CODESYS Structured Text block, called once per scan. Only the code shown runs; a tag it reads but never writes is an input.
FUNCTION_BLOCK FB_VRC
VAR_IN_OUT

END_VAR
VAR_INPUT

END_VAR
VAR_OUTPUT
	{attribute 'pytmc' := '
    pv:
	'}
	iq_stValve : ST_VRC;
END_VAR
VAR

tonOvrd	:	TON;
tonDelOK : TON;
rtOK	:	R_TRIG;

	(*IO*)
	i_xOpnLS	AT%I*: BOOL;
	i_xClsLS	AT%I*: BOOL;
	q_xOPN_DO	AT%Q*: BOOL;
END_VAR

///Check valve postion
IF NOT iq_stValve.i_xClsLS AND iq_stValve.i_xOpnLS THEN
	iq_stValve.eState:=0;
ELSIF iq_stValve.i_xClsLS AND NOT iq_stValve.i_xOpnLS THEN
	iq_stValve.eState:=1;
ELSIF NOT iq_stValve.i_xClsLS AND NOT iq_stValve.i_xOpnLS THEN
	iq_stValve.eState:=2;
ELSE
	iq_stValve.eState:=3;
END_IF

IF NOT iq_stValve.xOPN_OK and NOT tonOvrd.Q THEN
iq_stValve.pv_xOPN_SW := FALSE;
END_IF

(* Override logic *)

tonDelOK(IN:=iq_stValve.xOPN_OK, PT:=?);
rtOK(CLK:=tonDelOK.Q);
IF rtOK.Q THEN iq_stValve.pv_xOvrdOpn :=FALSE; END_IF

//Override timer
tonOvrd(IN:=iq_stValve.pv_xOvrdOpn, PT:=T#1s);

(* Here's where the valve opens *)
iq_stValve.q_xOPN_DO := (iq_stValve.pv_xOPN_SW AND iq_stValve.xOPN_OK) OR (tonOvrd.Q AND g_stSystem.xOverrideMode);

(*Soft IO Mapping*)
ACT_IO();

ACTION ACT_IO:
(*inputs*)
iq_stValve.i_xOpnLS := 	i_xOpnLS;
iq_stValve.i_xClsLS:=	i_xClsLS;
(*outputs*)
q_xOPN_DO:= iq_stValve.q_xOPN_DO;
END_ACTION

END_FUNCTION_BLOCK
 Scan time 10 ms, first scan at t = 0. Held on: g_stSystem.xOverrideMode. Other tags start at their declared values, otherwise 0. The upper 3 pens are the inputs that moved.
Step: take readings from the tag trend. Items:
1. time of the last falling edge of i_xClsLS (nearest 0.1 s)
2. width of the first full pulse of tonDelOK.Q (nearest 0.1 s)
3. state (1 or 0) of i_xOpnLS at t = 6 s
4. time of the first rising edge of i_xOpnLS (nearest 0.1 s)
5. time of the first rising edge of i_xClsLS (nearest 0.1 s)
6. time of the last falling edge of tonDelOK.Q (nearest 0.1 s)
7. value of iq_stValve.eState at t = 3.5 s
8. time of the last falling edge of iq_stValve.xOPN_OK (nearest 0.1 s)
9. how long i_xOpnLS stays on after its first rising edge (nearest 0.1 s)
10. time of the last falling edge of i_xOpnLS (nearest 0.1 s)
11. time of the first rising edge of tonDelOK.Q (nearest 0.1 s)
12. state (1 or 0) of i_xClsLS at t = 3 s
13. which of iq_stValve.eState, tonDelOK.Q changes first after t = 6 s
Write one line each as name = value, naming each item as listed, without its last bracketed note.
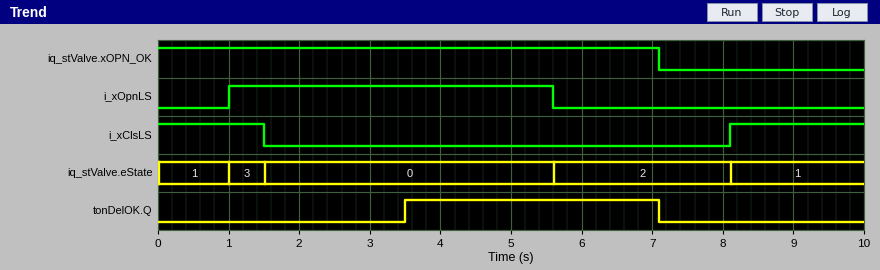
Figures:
time of the last falling edge of i_xClsLS = 1.5 s
width of the first full pulse of tonDelOK.Q = 3.6 s
state (1 or 0) of i_xOpnLS at t = 6 s = 0
time of the first rising edge of i_xOpnLS = 1.0 s
time of the first rising edge of i_xClsLS = 8.1 s
time of the last falling edge of tonDelOK.Q = 7.1 s
value of iq_stValve.eState at t = 3.5 s = 0
time of the last falling edge of iq_stValve.xOPN_OK = 7.1 s
how long i_xOpnLS stays on after its first rising edge = 4.6 s
time of the last falling edge of i_xOpnLS = 5.6 s
time of the first rising edge of tonDelOK.Q = 3.5 s
state (1 or 0) of i_xClsLS at t = 3 s = 0
which of iq_stValve.eState, tonDelOK.Q changes first after t = 6 s = tonDelOK.Q
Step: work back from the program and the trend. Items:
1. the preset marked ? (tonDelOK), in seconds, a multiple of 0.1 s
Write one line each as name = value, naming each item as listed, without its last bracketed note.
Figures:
the preset marked ? (tonDelOK), in seconds, a multiple of 0.1 s = 3.5 s
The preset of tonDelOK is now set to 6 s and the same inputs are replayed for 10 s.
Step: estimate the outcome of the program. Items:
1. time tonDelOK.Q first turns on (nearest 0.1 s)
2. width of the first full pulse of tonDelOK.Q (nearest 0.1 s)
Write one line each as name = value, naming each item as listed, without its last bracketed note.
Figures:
time tonDelOK.Q first turns on = 6.0 s
width of the first full pulse of tonDelOK.Q = 1.1 s
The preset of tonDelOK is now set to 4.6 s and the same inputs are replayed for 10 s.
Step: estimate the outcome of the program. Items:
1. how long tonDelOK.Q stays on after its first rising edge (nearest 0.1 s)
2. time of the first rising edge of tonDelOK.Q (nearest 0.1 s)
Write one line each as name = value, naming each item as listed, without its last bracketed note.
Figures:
how long tonDelOK.Q stays on after its first rising edge = 2.5 s
time of the first rising edge of tonDelOK.Q = 4.6 s
